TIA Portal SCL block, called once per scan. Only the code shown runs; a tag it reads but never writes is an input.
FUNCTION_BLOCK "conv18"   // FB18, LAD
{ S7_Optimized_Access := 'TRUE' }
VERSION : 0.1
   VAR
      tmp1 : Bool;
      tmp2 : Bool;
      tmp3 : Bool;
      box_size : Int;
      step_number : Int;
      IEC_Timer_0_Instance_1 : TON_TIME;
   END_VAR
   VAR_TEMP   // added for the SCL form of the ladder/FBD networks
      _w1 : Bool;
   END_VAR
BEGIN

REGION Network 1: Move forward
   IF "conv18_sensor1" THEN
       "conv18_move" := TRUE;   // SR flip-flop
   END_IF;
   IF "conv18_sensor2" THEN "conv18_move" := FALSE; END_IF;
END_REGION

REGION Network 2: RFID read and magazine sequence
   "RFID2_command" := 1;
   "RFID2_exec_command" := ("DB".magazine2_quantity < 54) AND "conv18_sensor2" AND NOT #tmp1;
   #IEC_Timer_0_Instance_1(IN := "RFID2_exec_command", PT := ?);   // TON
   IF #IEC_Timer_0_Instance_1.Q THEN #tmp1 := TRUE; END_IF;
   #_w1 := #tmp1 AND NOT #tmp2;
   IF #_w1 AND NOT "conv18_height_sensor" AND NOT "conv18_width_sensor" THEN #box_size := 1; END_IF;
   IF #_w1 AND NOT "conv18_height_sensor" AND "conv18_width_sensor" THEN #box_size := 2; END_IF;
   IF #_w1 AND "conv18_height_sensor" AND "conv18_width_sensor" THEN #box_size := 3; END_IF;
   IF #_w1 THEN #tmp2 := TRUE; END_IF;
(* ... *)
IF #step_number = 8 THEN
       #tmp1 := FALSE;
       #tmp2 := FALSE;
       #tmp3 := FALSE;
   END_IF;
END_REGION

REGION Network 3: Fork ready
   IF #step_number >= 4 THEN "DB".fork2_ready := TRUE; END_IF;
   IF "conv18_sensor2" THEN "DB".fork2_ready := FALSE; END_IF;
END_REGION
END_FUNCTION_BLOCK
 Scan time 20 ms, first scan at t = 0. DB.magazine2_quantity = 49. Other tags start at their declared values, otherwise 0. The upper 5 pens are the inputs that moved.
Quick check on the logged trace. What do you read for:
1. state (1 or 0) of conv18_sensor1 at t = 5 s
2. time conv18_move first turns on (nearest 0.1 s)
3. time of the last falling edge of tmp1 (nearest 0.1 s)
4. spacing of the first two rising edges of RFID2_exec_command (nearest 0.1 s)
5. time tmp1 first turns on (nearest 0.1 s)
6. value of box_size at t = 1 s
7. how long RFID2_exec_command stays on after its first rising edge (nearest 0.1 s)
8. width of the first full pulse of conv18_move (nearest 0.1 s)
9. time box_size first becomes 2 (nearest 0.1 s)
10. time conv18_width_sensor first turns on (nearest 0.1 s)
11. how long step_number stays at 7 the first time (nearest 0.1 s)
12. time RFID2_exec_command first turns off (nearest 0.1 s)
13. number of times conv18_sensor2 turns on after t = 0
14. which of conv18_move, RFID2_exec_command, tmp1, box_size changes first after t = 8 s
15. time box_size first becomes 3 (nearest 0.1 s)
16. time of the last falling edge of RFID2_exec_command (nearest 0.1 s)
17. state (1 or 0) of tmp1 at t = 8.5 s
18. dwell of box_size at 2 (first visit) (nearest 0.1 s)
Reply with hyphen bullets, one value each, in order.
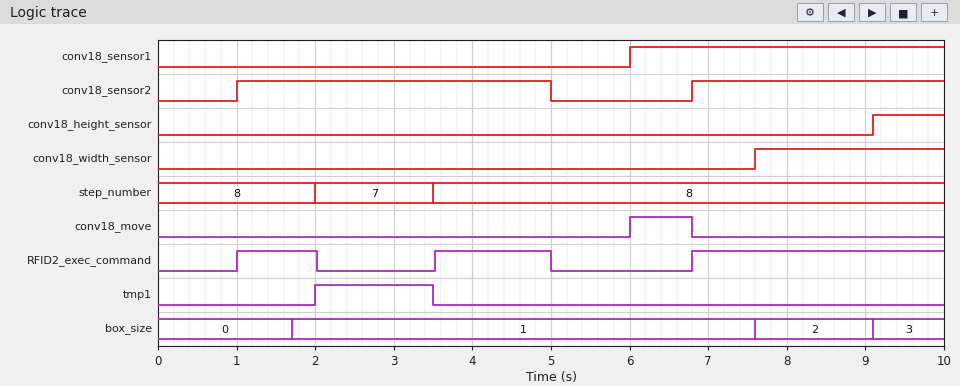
- 0
- 6.0 s
- 3.5 s
- 2.5 s
- 2.0 s
- 0
- 1.0 s
- 0.8 s
- 7.6 s
- 7.6 s
- 1.5 s
- 2.0 s
- 2
- box_size
- 9.1 s
- 5.0 s
- 0
- 1.5 s
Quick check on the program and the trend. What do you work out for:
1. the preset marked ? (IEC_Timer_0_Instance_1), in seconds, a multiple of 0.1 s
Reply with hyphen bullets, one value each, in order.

- 0.7 s
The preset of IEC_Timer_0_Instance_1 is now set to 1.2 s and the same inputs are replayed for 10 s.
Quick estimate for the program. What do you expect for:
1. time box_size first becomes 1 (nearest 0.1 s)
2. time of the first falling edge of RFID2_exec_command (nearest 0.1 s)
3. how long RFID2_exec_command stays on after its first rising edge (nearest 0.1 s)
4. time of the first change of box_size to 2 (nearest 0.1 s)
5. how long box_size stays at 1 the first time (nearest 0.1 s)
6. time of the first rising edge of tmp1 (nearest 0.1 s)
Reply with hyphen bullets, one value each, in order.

- 2.2 s
- 2.2 s
- 1.2 s
- 8.0 s
- 5.8 s
- 2.2 s
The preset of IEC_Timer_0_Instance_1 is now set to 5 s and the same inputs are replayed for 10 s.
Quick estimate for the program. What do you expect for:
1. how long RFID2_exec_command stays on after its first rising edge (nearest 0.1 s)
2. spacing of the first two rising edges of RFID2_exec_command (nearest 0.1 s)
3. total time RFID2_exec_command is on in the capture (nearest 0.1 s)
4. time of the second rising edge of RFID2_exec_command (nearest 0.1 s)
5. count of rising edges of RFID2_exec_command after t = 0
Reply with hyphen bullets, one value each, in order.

- 4.0 s
- 5.8 s
- 7.2 s
- 6.8 s
- 2
